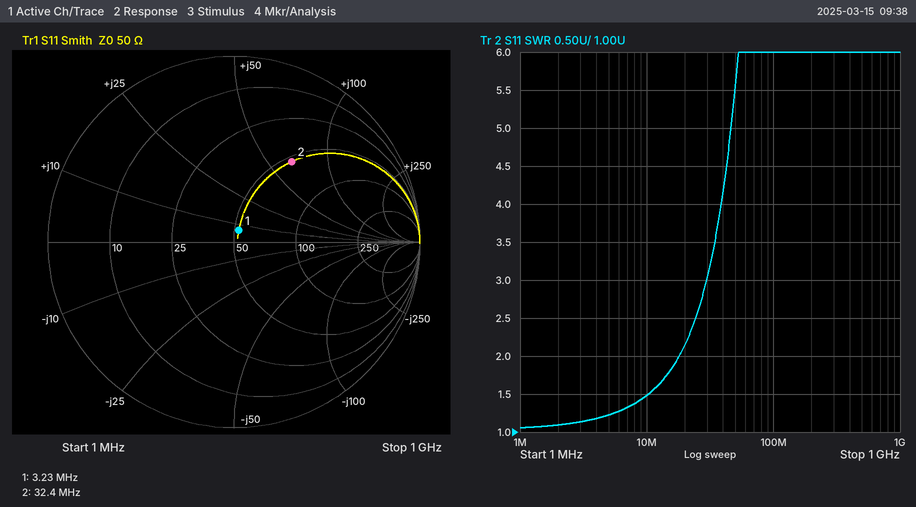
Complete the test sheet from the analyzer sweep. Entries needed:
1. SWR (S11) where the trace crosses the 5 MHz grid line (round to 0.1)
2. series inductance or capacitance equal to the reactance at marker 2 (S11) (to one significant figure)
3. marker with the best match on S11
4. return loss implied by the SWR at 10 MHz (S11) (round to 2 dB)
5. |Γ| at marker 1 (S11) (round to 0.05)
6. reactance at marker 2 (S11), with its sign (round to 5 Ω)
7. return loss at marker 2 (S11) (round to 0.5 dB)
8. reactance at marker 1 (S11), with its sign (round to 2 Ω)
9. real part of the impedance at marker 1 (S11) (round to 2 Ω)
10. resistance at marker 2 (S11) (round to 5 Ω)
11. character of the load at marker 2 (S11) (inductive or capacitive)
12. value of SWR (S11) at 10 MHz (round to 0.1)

1.2
300 nH
marker 1
14 dB
0.05
+65 Ω
5.5 dB
+6 Ω
52 Ω
55 Ω
inductive
1.5
